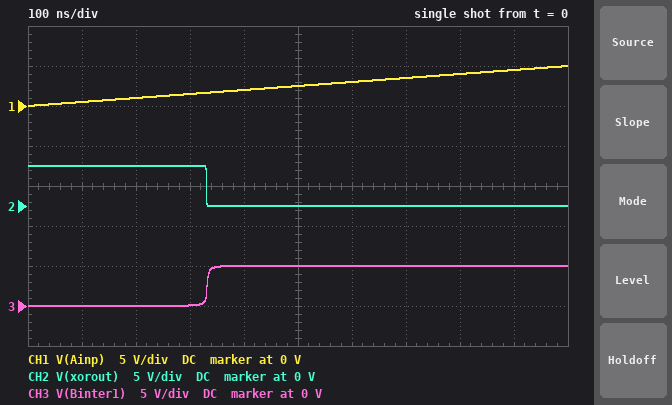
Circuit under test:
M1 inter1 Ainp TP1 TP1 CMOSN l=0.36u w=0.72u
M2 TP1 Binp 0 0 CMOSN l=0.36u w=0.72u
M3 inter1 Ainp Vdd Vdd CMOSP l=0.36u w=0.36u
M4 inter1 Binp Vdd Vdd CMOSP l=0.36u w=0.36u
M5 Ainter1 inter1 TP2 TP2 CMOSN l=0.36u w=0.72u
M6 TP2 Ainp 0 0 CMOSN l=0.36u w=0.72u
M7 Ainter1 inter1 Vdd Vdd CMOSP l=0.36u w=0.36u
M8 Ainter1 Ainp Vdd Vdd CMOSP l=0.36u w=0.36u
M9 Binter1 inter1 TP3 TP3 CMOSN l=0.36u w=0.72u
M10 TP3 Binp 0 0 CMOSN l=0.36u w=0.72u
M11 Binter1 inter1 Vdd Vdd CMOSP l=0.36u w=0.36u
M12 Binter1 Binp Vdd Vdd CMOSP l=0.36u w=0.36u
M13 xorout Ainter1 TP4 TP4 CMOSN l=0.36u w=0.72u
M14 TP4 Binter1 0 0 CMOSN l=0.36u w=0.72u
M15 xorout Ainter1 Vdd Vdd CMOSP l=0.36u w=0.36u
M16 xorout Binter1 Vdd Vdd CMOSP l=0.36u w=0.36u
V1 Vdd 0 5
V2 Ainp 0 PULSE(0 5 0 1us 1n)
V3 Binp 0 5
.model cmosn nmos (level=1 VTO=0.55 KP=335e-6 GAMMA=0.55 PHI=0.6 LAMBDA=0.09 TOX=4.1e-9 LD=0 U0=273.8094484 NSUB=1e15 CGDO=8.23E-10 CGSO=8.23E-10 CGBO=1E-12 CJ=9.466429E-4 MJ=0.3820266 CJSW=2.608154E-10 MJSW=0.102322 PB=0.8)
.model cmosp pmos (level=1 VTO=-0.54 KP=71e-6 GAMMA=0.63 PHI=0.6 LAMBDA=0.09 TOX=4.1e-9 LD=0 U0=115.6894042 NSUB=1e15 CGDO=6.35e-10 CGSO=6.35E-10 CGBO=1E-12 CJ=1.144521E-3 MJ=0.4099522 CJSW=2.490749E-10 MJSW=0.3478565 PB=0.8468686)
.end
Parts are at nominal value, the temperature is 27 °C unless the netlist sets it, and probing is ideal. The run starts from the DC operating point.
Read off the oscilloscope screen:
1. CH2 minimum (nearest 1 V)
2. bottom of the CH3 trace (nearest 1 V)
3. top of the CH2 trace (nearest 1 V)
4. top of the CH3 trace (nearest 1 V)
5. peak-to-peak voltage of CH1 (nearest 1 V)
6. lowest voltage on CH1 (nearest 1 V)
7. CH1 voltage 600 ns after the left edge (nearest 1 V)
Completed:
0 V
0 V
5 V
5 V
5 V
0 V
3 V
